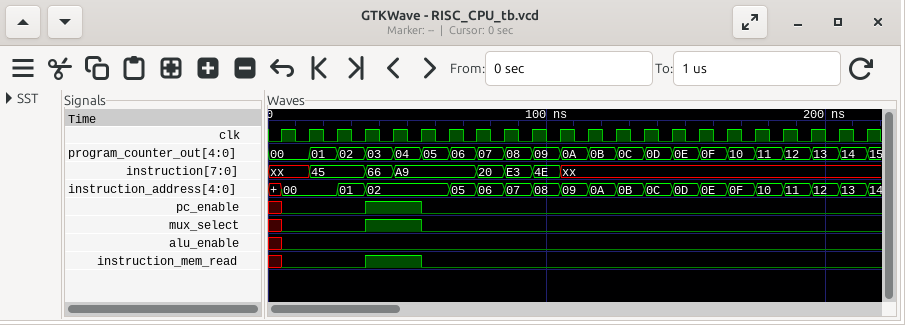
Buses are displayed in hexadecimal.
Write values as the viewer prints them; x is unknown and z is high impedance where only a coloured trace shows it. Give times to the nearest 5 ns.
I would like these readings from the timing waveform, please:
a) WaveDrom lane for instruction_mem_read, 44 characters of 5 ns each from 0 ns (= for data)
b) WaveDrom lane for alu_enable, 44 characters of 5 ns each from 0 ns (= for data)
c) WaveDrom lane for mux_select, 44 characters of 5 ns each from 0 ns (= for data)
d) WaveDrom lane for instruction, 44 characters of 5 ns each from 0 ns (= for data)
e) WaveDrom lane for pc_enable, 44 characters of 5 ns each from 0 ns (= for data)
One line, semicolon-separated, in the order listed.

{name: 'instruction_mem_read', wave: 'x0.....1...0................................'}; {name: 'alu_enable', wave: 'x0..........................................'}; {name: 'mux_select', wave: 'x0.....1...0................................'}; {name: 'instruction', wave: 'x..=...=.=.....=.=.=.x......................', data: '45 66 A9 20 E3 4E'}; {name: 'pc_enable', wave: 'x0.....1...0................................'}
